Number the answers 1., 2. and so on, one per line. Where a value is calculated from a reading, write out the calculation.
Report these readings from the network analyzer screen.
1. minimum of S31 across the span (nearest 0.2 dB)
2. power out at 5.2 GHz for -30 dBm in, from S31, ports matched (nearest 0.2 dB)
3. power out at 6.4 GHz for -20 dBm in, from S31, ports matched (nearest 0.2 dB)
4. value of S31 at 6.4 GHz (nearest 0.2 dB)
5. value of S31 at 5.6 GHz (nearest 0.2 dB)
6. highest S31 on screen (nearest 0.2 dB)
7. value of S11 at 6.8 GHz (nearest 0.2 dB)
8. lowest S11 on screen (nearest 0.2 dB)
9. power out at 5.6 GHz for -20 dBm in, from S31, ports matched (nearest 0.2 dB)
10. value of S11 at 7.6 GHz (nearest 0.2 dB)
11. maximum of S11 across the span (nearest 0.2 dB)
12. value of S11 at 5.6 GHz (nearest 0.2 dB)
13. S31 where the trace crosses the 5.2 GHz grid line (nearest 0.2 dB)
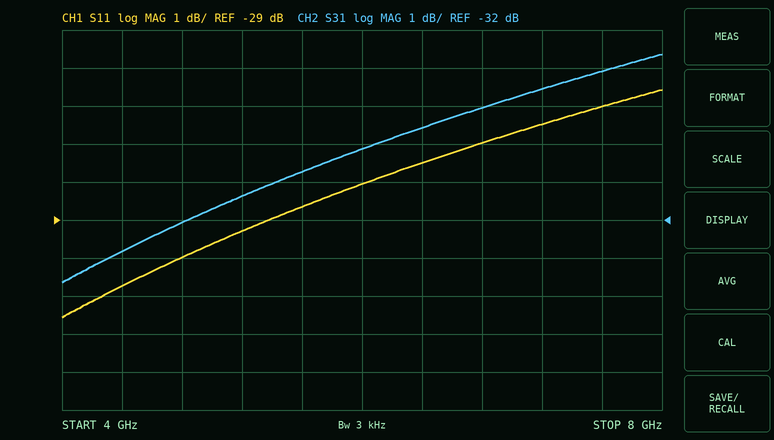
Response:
1. -33.6 dB
2. -30 dBm + (-31.4 dB) = -61.4 dBm
3. -20 dBm + (-29.6 dB) = -49.6 dBm
4. -29.6 dB
5. -30.8 dB
6. -27.6 dB
7. -27.0 dB
8. -31.6 dB
9. -20 dBm + (-30.8 dB) = -50.8 dBm
10. -26.0 dB
11. -25.6 dB
12. -28.6 dB
13. -31.4 dB
